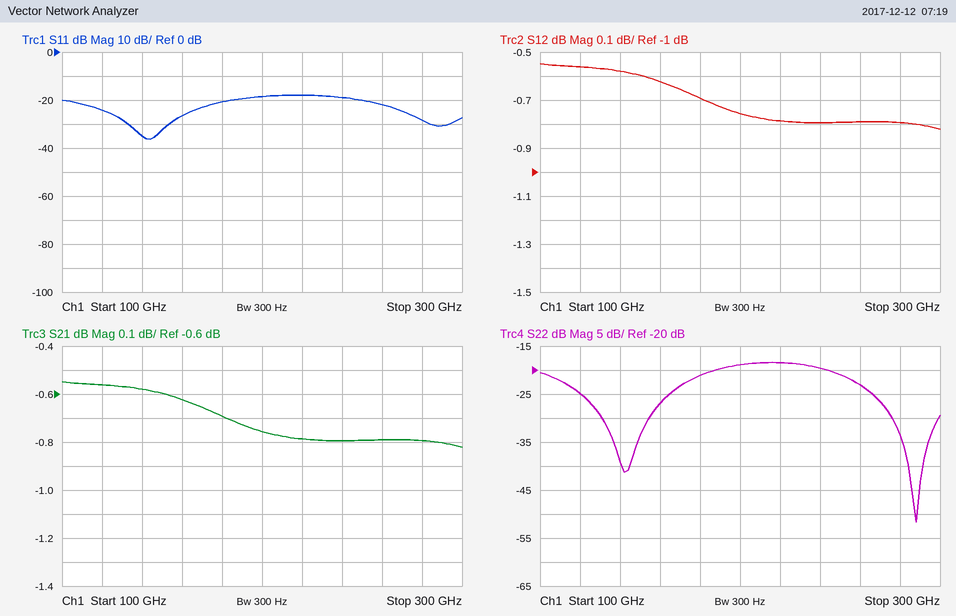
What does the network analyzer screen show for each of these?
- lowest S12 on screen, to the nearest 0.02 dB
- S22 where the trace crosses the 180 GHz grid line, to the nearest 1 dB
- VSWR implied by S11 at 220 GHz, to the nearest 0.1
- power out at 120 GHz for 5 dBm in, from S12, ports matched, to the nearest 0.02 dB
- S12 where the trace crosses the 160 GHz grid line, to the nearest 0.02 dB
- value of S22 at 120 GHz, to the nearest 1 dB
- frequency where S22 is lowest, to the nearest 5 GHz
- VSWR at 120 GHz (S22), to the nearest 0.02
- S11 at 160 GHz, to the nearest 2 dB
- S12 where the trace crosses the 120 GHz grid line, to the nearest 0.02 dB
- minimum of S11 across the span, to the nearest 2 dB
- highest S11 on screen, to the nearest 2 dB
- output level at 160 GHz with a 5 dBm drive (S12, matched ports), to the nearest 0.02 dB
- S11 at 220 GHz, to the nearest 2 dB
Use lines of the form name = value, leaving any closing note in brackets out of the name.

lowest S12 on screen, to the nearest 0.02 dB = -0.82 dB
S22 where the trace crosses the 180 GHz grid line, to the nearest 1 dB = -21 dB
VSWR implied by S11 at 220 GHz, to the nearest 0.1 = 1.3
power out at 120 GHz for 5 dBm in, from S12, ports matched, to the nearest 0.02 dB = 4.44 dBm
S12 where the trace crosses the 160 GHz grid line, to the nearest 0.02 dB = -0.62 dB
value of S22 at 120 GHz, to the nearest 1 dB = -25 dB
frequency where S22 is lowest, to the nearest 5 GHz = 290 GHz
VSWR at 120 GHz (S22), to the nearest 0.02 = 1.12
S11 at 160 GHz, to the nearest 2 dB = -26 dB
S12 where the trace crosses the 120 GHz grid line, to the nearest 0.02 dB = -0.56 dB
minimum of S11 across the span, to the nearest 2 dB = -36 dB
highest S11 on screen, to the nearest 2 dB = -18 dB
output level at 160 GHz with a 5 dBm drive (S12, matched ports), to the nearest 0.02 dB = 4.38 dBm
S11 at 220 GHz, to the nearest 2 dB = -18 dB
